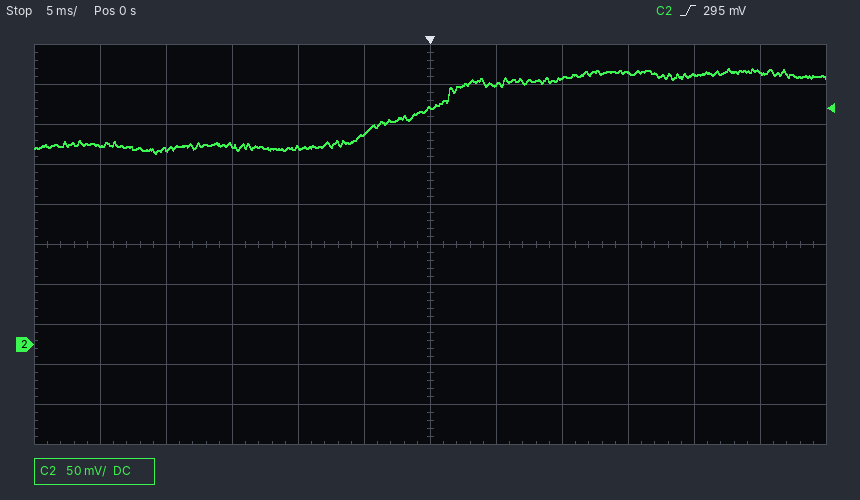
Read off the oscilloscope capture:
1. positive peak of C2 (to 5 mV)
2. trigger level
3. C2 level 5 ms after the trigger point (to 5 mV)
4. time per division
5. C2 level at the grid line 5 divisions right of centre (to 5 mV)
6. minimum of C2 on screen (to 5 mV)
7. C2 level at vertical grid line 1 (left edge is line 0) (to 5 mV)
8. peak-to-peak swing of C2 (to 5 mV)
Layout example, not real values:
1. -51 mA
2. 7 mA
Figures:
1. 345 mV
2. 295 mV
3. 325 mV
4. 5 ms
5. 340 mV
6. 240 mV
7. 250 mV
8. 105 mV
